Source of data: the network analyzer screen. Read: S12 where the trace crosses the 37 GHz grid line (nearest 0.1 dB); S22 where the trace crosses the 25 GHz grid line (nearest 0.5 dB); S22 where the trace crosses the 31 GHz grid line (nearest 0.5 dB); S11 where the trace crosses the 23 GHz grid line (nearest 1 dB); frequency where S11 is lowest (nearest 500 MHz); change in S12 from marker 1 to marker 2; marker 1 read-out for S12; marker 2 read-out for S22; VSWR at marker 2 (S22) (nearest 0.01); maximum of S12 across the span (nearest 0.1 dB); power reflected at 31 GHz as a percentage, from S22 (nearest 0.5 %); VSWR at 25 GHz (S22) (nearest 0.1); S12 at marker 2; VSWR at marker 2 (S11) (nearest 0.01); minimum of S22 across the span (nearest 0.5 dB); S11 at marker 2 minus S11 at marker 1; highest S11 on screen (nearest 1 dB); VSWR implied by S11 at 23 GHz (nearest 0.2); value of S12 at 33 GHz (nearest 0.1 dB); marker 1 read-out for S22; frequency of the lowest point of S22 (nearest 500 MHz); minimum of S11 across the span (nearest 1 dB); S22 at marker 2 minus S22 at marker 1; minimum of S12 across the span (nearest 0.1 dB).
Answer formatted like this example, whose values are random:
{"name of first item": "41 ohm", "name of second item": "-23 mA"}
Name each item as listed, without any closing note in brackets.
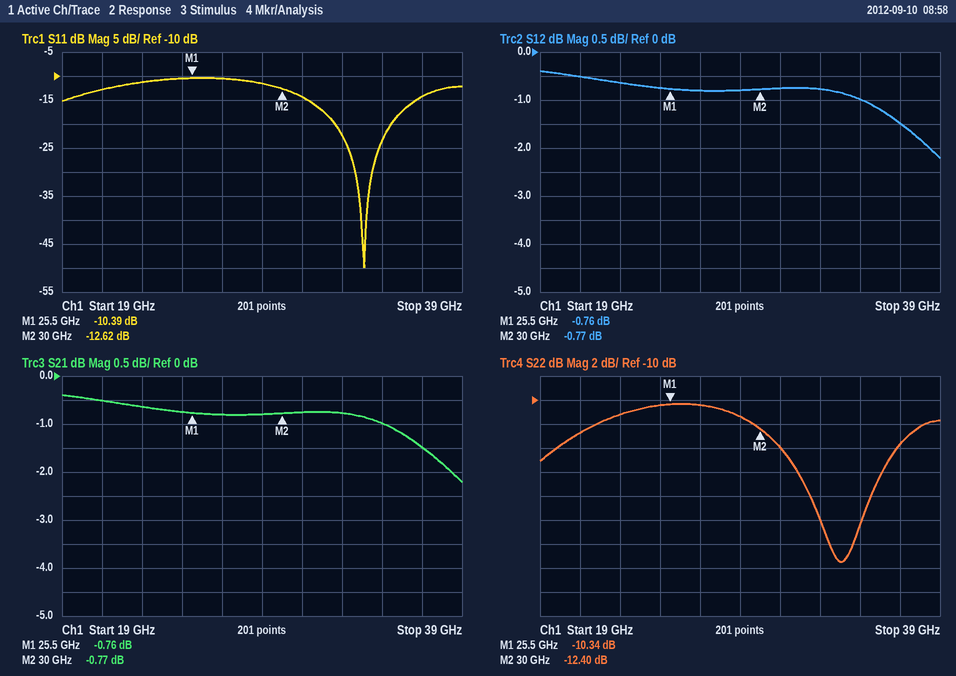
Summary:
{"S12 where the trace crosses the 37 GHz grid line": "-1.5 dB", "S22 where the trace crosses the 25 GHz grid line": "-10.5 dB", "S22 where the trace crosses the 31 GHz grid line": "-14.0 dB", "S11 where the trace crosses the 23 GHz grid line": "-11 dB", "frequency where S11 is lowest": "34.0 GHz", "change in S12 from marker 1 to marker 2": "-0.01 dB", "marker 1 read-out for S12": "-0.76 dB", "marker 2 read-out for S22": "-12.40 dB", "VSWR at marker 2 (S22)": "1.63", "maximum of S12 across the span": "-0.4 dB", "power reflected at 31 GHz as a percentage, from S22": "4.0 %", "VSWR at 25 GHz (S22)": "1.9", "S12 at marker 2": "-0.77 dB", "VSWR at marker 2 (S11)": "1.61", "minimum of S22 across the span": "-23.5 dB", "S11 at marker 2 minus S11 at marker 1": "-2.23 dB", "highest S11 on screen": "-10 dB", "VSWR implied by S11 at 23 GHz": "1.8", "value of S12 at 33 GHz": "-0.8 dB", "marker 1 read-out for S22": "-10.34 dB", "frequency of the lowest point of S22": "34.0 GHz", "minimum of S11 across the span": "-50 dB", "S22 at marker 2 minus S22 at marker 1": "-2.06 dB", "minimum of S12 across the span": "-2.2 dB"}
